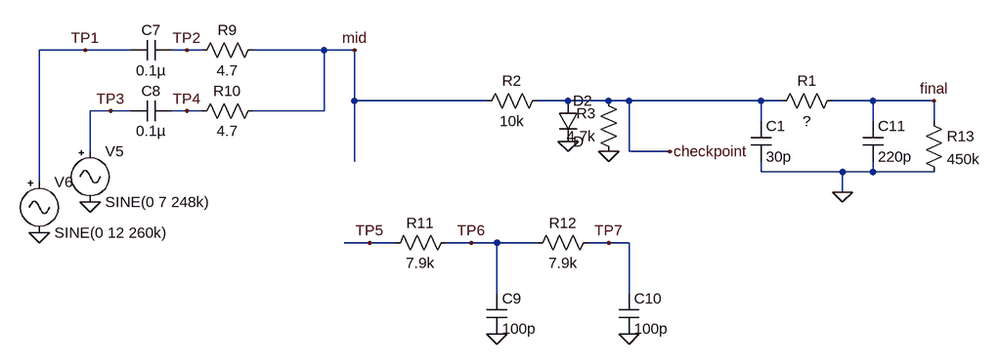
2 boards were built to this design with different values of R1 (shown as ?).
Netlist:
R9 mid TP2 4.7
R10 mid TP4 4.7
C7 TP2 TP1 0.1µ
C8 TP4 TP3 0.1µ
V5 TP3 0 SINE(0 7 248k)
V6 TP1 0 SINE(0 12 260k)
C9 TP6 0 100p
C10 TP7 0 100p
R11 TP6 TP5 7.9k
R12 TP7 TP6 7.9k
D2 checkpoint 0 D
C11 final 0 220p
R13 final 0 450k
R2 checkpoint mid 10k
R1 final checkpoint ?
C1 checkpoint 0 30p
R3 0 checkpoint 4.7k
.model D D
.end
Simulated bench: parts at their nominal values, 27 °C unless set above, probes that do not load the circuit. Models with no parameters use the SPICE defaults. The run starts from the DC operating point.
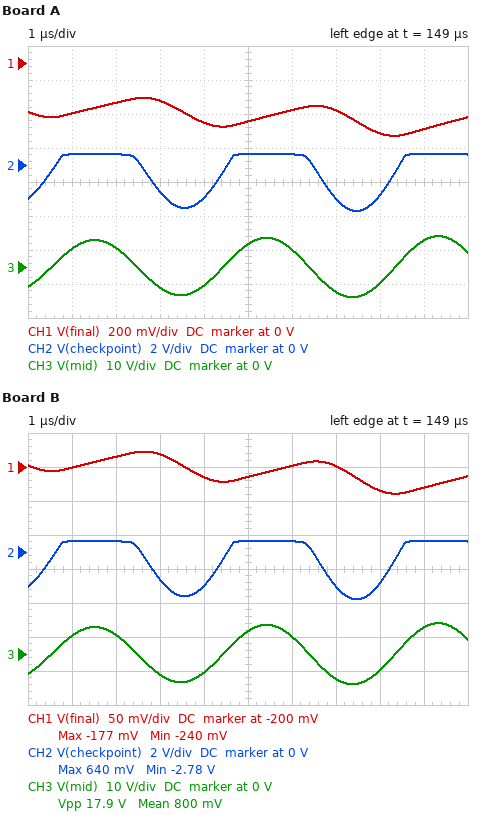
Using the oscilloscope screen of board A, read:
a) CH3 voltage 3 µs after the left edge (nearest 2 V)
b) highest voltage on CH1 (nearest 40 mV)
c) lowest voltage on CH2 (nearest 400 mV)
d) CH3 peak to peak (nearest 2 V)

-6 V
-200 mV
-2.8 V
18 V
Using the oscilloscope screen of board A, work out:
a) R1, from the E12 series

68 kΩ
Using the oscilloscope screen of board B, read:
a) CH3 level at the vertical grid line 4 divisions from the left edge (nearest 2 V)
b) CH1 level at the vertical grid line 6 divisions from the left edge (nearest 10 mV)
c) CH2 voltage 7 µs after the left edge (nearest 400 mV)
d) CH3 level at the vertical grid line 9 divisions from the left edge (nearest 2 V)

-6 V
-200 mV
-2.0 V
8 V
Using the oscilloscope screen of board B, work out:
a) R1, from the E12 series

270 kΩ
